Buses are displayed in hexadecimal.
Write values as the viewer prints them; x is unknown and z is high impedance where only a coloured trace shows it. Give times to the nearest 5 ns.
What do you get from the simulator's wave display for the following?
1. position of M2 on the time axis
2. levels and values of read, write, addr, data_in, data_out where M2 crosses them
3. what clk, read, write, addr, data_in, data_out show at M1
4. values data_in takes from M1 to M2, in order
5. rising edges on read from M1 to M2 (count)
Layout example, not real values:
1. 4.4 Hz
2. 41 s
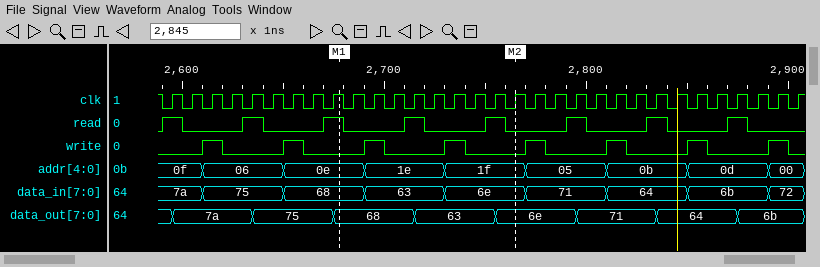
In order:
1. 2765 ns
2. read=0, write=0, addr=1f, data_in=6e, data_out=6e
3. clk=1, read=1, write=0, addr=0e, data_in=68, data_out=68
4. 68, 63, 6e
5. 2
